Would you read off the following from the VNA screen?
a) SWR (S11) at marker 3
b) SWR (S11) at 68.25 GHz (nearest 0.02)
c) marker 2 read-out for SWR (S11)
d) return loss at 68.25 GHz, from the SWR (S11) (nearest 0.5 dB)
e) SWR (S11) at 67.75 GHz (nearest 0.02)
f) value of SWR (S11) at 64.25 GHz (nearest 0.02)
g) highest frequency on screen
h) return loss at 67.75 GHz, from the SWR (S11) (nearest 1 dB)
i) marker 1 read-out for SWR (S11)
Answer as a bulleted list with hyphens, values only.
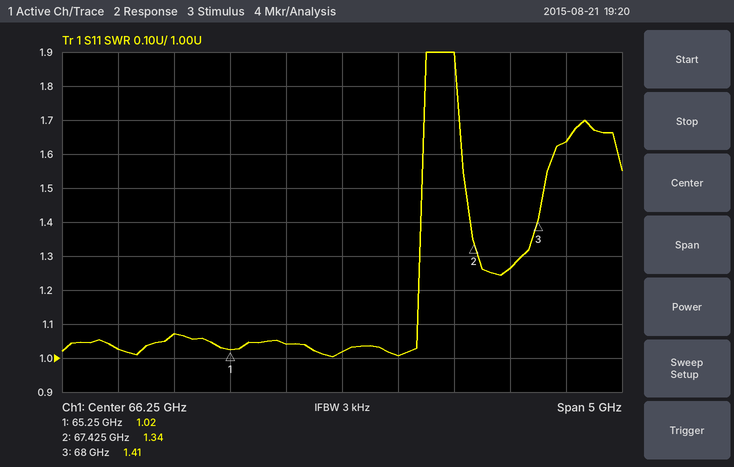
- 1.41
- 1.64
- 1.34
- 12.5 dB
- 1.26
- 1.02
- 68.75 GHz
- 19 dB
- 1.02
